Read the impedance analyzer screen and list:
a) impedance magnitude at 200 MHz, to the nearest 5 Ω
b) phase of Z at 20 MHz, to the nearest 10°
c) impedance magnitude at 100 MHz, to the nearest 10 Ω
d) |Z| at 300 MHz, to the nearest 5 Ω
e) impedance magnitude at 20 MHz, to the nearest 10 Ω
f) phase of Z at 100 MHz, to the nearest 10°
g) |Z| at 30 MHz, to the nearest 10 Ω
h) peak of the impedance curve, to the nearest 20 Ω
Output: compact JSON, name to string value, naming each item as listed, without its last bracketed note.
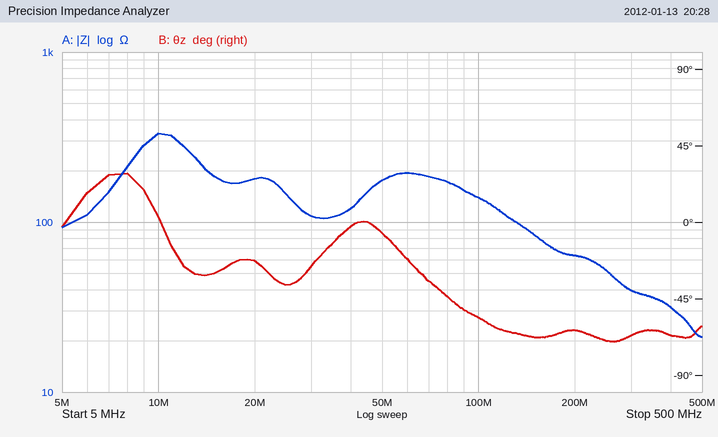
{"impedance magnitude at 200 MHz, to the nearest 5 Ω": "65 Ω", "phase of Z at 20 MHz, to the nearest 10°": "-20°", "impedance magnitude at 100 MHz, to the nearest 10 Ω": "140 Ω", "|Z| at 300 MHz, to the nearest 5 Ω": "40 Ω", "impedance magnitude at 20 MHz, to the nearest 10 Ω": "180 Ω", "phase of Z at 100 MHz, to the nearest 10°": "-60°", "|Z| at 30 MHz, to the nearest 10 Ω": "110 Ω", "peak of the impedance curve, to the nearest 20 Ω": "340 Ω"}
